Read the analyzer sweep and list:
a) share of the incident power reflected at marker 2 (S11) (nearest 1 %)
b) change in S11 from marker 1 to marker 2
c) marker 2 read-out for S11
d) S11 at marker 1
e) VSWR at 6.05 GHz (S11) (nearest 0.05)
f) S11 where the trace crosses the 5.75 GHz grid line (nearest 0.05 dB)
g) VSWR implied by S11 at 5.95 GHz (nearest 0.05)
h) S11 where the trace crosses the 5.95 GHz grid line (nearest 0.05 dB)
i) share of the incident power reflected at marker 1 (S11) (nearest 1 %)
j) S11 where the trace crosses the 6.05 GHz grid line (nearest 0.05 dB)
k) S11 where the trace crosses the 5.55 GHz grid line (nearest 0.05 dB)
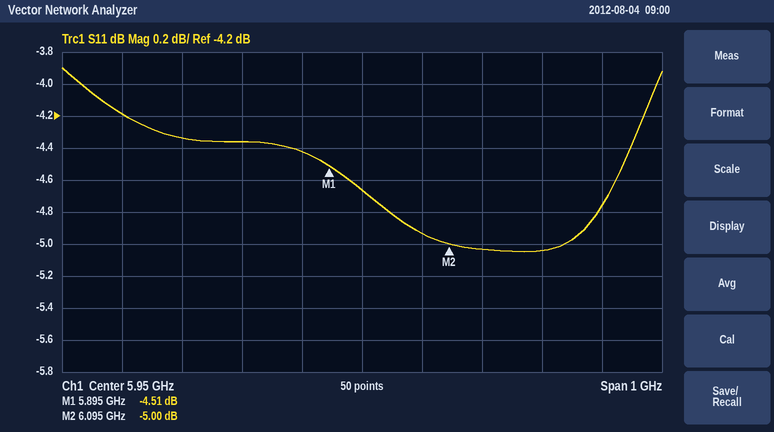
32 %
-0.49 dB
-5.00 dB
-4.51 dB
3.60
-4.35 dB
3.80
-4.65 dB
35 %
-4.95 dB
-4.20 dB
